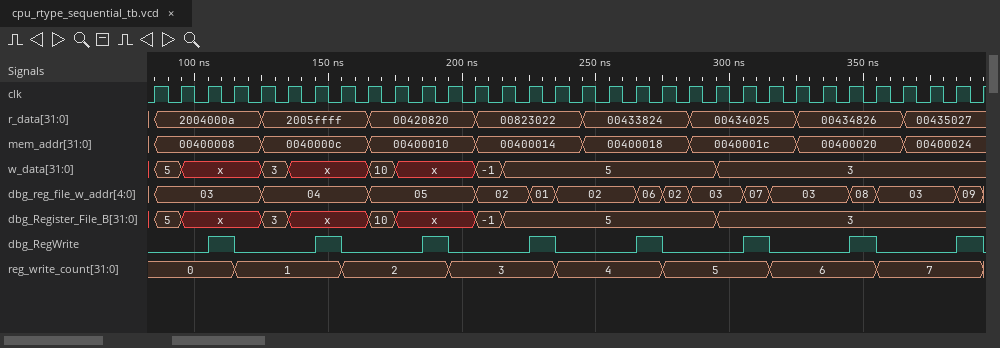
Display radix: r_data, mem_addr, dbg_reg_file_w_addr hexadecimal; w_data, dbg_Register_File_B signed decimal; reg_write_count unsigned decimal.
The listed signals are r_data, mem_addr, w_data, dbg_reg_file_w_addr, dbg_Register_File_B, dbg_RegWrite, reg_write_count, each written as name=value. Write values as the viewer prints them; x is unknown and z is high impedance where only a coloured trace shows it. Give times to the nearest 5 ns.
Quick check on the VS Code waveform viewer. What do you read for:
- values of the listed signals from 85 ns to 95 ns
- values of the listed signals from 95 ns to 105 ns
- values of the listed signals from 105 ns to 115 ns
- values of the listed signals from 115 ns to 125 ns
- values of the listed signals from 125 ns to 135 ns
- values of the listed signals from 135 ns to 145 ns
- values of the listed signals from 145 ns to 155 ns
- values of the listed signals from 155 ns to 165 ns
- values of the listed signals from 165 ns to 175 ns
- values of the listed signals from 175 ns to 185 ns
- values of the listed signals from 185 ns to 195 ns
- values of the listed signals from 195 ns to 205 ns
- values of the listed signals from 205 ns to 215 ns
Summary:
r_data=2004000a, mem_addr=00400008, w_data=5, dbg_reg_file_w_addr=03, dbg_Register_File_B=5, dbg_RegWrite=0, reg_write_count=0
r_data=2004000a, mem_addr=00400008, w_data=x, dbg_reg_file_w_addr=03, dbg_Register_File_B=x, dbg_RegWrite=0, reg_write_count=0
r_data=2004000a, mem_addr=00400008, w_data=x, dbg_reg_file_w_addr=03, dbg_Register_File_B=x, dbg_RegWrite=1, reg_write_count=0
r_data=2004000a, mem_addr=00400008, w_data=x, dbg_reg_file_w_addr=03, dbg_Register_File_B=x, dbg_RegWrite=0, reg_write_count=1
r_data=2005ffff, mem_addr=0040000c, w_data=3, dbg_reg_file_w_addr=04, dbg_Register_File_B=3, dbg_RegWrite=0, reg_write_count=1
r_data=2005ffff, mem_addr=0040000c, w_data=x, dbg_reg_file_w_addr=04, dbg_Register_File_B=x, dbg_RegWrite=0, reg_write_count=1
r_data=2005ffff, mem_addr=0040000c, w_data=x, dbg_reg_file_w_addr=04, dbg_Register_File_B=x, dbg_RegWrite=1, reg_write_count=1
r_data=2005ffff, mem_addr=0040000c, w_data=x, dbg_reg_file_w_addr=04, dbg_Register_File_B=x, dbg_RegWrite=0, reg_write_count=2
r_data=00420820, mem_addr=00400010, w_data=10, dbg_reg_file_w_addr=05, dbg_Register_File_B=10, dbg_RegWrite=0, reg_write_count=2
r_data=00420820, mem_addr=00400010, w_data=x, dbg_reg_file_w_addr=05, dbg_Register_File_B=x, dbg_RegWrite=0, reg_write_count=2
r_data=00420820, mem_addr=00400010, w_data=x, dbg_reg_file_w_addr=05, dbg_Register_File_B=x, dbg_RegWrite=1, reg_write_count=2
r_data=00420820, mem_addr=00400010, w_data=x, dbg_reg_file_w_addr=05, dbg_Register_File_B=x, dbg_RegWrite=0, reg_write_count=3
r_data=00823022, mem_addr=00400014, w_data=-1, dbg_reg_file_w_addr=02, dbg_Register_File_B=-1, dbg_RegWrite=0, reg_write_count=3
